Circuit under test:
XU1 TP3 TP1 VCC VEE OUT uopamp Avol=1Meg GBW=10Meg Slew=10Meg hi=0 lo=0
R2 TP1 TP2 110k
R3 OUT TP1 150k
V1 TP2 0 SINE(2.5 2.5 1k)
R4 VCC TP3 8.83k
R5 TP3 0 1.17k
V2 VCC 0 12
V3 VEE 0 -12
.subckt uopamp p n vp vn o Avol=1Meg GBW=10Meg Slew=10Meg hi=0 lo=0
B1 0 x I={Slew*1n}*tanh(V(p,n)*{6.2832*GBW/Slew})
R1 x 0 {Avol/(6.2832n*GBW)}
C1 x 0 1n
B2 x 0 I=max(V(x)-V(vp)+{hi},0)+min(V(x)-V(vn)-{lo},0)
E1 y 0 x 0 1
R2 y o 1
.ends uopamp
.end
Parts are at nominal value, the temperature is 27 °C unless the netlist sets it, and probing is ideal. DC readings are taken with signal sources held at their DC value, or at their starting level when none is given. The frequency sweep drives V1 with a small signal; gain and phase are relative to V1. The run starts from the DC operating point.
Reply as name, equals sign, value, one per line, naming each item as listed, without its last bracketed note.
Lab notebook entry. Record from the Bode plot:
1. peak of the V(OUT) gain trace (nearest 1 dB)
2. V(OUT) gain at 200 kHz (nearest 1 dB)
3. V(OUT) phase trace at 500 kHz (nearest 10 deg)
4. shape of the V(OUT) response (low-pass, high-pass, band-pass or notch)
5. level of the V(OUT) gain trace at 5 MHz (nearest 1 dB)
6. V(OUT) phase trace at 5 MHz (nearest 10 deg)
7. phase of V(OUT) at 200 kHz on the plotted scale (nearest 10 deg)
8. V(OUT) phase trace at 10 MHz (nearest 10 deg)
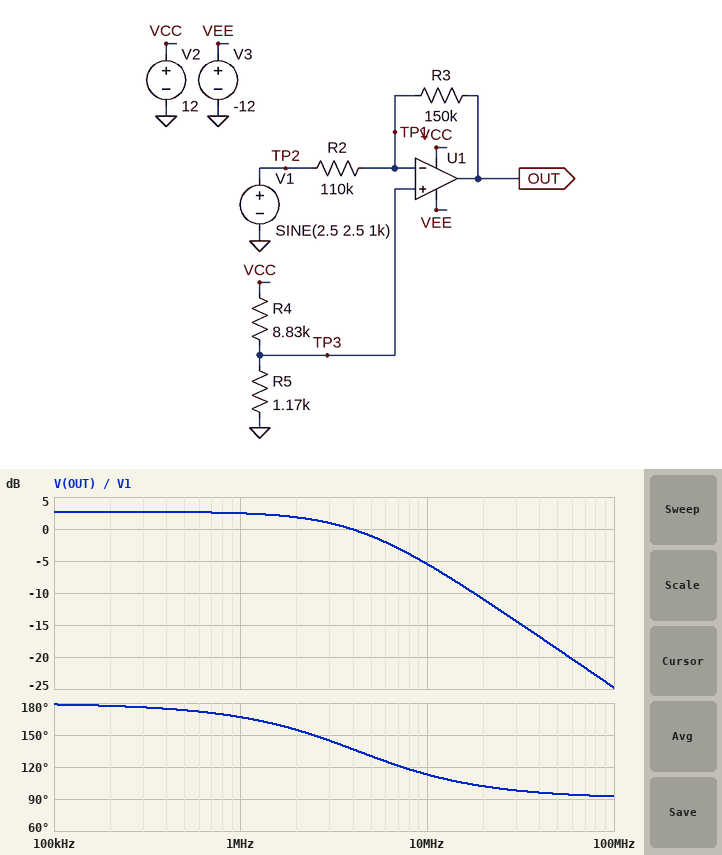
peak of the V(OUT) gain trace = 3 dB
V(OUT) gain at 200 kHz = 3 dB
V(OUT) phase trace at 500 kHz = 170 deg
shape of the V(OUT) response = low-pass
level of the V(OUT) gain trace at 5 MHz = -1 dB
V(OUT) phase trace at 5 MHz = 130 deg
phase of V(OUT) at 200 kHz on the plotted scale = 180 deg
V(OUT) phase trace at 10 MHz = 110 deg
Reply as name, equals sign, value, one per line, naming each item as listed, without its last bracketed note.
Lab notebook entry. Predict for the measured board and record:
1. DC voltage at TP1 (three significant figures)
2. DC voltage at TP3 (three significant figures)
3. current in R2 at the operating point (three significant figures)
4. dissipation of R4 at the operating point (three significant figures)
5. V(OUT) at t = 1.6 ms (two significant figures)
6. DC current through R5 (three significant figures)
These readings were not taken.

DC voltage at TP1 = 1.40 V
DC voltage at TP3 = 1.40 V
current in R2 at the operating point = 9.96 µA
dissipation of R4 at the operating point = 12.7 mW
V(OUT) at t = 1.6 ms = 1.9 V
DC current through R5 = 1.20 mA
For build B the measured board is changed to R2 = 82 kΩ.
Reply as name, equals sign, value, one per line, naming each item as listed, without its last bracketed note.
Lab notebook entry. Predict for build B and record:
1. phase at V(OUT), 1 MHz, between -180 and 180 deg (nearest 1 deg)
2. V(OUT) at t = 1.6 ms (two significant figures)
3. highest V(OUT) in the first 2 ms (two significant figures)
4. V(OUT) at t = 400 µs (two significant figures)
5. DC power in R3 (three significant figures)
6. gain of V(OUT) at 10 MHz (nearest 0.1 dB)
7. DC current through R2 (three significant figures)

phase at V(OUT), 1 MHz, between -180 and 180 deg = 164 deg
V(OUT) at t = 1.6 ms = 2.1 V
highest V(OUT) in the first 2 ms = 4.0 V
V(OUT) at t = 400 µs = -3.3 V
DC power in R3 = 26.8 µW
gain of V(OUT) at 10 MHz = -4.3 dB
DC current through R2 = 13.4 µA
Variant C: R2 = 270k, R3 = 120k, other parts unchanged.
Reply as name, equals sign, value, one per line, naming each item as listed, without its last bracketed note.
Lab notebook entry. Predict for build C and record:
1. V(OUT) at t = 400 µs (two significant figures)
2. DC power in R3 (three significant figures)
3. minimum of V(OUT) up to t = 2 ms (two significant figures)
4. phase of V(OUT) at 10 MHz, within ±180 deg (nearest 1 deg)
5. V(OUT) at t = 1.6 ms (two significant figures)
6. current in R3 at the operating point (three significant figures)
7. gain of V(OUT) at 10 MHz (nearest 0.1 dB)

V(OUT) at t = 400 µs = 260 mV
DC power in R3 = 1.98 µW
minimum of V(OUT) up to t = 2 ms = -190 mV
phase of V(OUT) at 10 MHz, within ±180 deg = 125 deg
V(OUT) at t = 1.6 ms = 1.6 V
current in R3 at the operating point = 4.06 µA
gain of V(OUT) at 10 MHz = -11.9 dB
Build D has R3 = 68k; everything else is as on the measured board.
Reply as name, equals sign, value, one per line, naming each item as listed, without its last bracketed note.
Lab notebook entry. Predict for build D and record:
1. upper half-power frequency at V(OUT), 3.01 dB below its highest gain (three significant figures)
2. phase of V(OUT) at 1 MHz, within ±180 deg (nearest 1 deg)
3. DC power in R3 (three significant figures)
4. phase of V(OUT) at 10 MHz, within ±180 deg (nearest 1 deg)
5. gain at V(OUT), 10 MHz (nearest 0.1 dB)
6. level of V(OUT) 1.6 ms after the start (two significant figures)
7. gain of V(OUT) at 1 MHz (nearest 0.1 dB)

upper half-power frequency at V(OUT), 3.01 dB below its highest gain = 6.18 MHz
phase of V(OUT) at 1 MHz, within ±180 deg = 171 deg
DC power in R3 = 6.75 µW
phase of V(OUT) at 10 MHz, within ±180 deg = 122 deg
gain at V(OUT), 10 MHz = -9.8 dB
level of V(OUT) 1.6 ms after the start = 1.6 V
gain of V(OUT) at 1 MHz = -4.3 dB
